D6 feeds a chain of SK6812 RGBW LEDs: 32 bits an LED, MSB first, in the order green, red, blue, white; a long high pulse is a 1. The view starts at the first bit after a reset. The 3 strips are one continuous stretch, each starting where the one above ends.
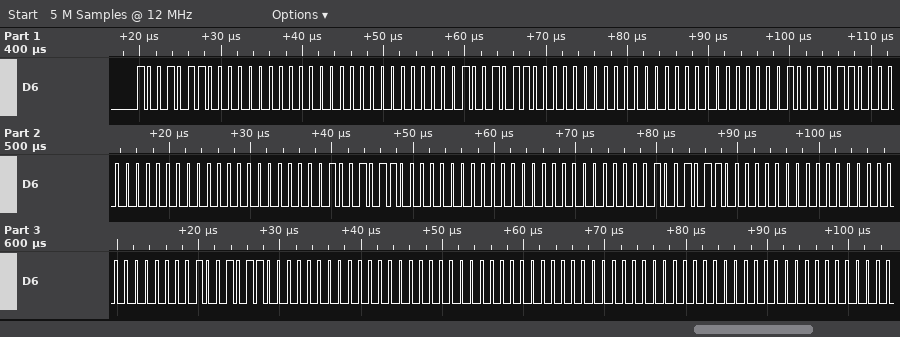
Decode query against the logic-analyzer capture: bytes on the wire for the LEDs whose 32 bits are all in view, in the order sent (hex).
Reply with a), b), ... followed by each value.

a) 96 00 00 00 96 00 00 00 96 00 00 00 96 00 00 00 96 00 00 00 96 00 00 00 00 00 00 00
